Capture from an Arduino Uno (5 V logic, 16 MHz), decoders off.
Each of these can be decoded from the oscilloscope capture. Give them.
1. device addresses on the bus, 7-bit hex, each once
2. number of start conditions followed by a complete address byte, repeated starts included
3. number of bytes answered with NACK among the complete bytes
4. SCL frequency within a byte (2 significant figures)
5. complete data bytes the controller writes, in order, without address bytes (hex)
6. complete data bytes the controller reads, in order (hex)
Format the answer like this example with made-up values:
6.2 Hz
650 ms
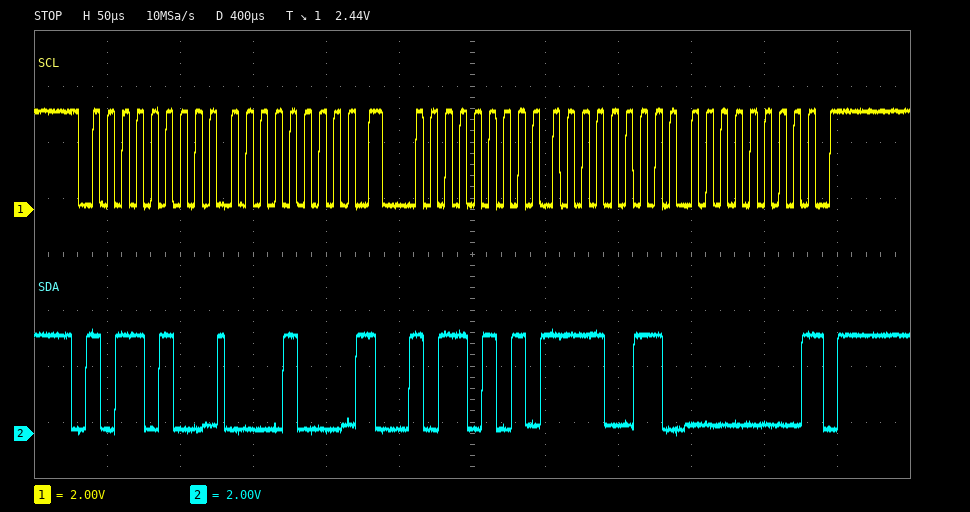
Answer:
0x5A
2
1
100 kHz
08
F3 00
